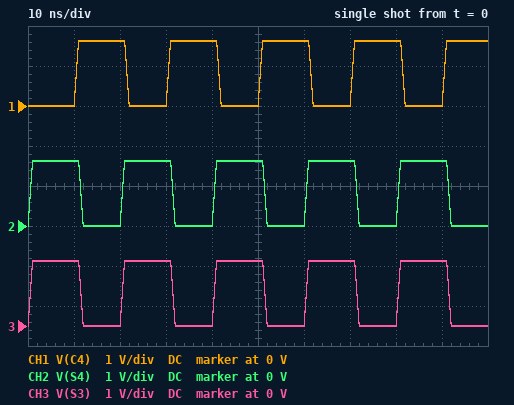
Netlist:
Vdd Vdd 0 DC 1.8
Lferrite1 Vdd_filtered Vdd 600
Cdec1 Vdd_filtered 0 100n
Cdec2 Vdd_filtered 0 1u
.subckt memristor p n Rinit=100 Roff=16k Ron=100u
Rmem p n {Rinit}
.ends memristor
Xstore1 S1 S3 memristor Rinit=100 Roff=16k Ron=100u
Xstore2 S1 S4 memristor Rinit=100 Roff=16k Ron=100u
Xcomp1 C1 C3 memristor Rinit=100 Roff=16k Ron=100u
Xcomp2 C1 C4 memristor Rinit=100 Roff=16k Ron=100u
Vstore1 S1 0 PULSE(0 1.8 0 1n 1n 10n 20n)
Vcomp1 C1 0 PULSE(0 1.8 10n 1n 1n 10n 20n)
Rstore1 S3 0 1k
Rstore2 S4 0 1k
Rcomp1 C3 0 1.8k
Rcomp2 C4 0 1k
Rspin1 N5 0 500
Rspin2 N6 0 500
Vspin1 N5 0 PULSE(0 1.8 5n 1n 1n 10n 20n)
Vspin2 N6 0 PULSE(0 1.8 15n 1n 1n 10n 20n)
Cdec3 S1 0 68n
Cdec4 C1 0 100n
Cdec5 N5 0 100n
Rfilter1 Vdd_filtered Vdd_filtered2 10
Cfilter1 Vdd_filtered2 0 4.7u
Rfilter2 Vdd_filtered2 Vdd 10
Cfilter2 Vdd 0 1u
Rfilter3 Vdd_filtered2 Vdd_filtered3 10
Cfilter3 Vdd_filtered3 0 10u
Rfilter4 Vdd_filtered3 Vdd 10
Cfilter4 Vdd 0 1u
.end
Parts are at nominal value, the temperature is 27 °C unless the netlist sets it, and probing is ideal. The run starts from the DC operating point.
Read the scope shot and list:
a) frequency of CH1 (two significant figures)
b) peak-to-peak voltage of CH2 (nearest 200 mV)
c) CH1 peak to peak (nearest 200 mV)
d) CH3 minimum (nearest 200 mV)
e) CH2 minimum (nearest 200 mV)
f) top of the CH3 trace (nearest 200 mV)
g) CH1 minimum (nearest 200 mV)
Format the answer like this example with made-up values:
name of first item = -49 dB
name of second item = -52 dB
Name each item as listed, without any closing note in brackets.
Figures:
frequency of CH1 = 50 MHz
peak-to-peak voltage of CH2 = 1.6 V
CH1 peak to peak = 1.6 V
CH3 minimum = 0 V
CH2 minimum = 0 V
top of the CH3 trace = 1.6 V
CH1 minimum = 0 V
